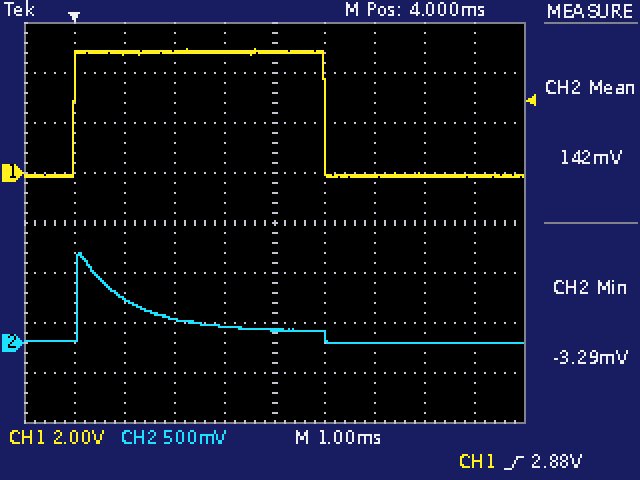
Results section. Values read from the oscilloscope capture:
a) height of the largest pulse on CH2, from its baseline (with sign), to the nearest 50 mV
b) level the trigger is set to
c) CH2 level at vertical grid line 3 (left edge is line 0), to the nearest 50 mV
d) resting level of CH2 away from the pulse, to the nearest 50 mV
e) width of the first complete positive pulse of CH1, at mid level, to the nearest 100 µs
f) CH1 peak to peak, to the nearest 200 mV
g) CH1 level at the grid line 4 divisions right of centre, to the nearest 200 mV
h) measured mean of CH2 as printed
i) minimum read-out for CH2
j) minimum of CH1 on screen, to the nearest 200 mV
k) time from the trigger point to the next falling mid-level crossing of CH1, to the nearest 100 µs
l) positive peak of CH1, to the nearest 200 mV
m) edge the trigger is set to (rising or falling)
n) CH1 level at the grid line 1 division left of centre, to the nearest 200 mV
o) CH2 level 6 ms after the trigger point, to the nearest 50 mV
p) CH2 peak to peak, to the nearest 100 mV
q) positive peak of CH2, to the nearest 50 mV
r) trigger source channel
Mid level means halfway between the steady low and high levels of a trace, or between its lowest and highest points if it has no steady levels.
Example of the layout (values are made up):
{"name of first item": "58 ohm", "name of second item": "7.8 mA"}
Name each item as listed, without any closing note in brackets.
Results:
{"height of the largest pulse on CH2, from its baseline (with sign), to the nearest 50 mV": "+900 mV", "level the trigger is set to": "2.88 V", "CH2 level at vertical grid line 3 (left edge is line 0), to the nearest 50 mV": "250 mV", "resting level of CH2 away from the pulse, to the nearest 50 mV": "0 mV", "width of the first complete positive pulse of CH1, at mid level, to the nearest 100 µs": "5.0 ms", "CH1 peak to peak, to the nearest 200 mV": "5.2 V", "CH1 level at the grid line 4 divisions right of centre, to the nearest 200 mV": "-200 mV", "measured mean of CH2 as printed": "142 mV", "minimum read-out for CH2": "-3.29 mV", "minimum of CH1 on screen, to the nearest 200 mV": "-200 mV", "time from the trigger point to the next falling mid-level crossing of CH1, to the nearest 100 µs": "5.0 ms", "positive peak of CH1, to the nearest 200 mV": "5.0 V", "edge the trigger is set to": "rising", "CH1 level at the grid line 1 division left of centre, to the nearest 200 mV": "4.8 V", "CH2 level 6 ms after the trigger point, to the nearest 50 mV": "0 mV", "CH2 peak to peak, to the nearest 100 mV": "900 mV", "positive peak of CH2, to the nearest 50 mV": "900 mV", "trigger source channel": "CH1"}
